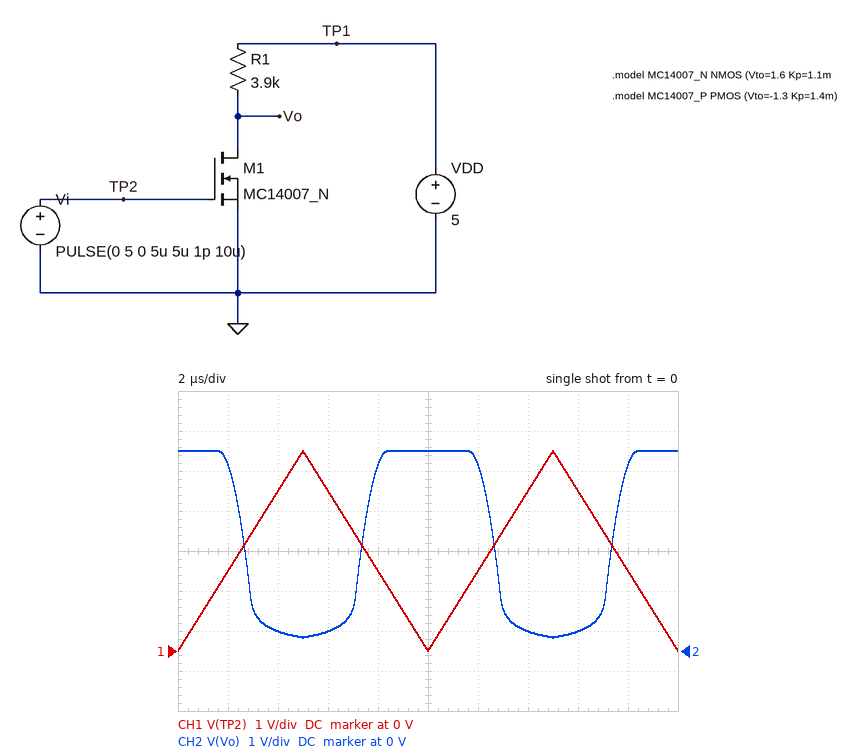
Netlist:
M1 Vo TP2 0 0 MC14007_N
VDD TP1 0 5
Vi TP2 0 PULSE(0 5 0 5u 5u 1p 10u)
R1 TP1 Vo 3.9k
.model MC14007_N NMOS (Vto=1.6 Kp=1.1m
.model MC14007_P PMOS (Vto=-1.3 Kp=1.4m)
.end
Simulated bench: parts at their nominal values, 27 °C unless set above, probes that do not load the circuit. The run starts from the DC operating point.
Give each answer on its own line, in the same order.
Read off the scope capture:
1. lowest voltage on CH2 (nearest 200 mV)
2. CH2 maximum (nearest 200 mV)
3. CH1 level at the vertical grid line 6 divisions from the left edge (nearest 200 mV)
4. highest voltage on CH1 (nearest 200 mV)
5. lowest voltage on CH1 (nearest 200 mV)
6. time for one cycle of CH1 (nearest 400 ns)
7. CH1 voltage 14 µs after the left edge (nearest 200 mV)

400 mV
5.0 V
2.0 V
5.0 V
0 V
10.0 µs
4.0 V
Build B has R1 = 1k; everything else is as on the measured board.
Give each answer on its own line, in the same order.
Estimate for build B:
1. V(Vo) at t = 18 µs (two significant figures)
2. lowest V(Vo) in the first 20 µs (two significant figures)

4.9 V
1.2 V
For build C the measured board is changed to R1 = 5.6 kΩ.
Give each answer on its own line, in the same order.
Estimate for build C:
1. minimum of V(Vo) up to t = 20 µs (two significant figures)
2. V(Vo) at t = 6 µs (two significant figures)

240 mV
340 mV
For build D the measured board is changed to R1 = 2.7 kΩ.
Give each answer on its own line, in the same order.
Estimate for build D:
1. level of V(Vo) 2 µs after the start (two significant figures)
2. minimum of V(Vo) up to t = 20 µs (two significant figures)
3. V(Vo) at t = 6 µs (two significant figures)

4.8 V
480 mV
710 mV
